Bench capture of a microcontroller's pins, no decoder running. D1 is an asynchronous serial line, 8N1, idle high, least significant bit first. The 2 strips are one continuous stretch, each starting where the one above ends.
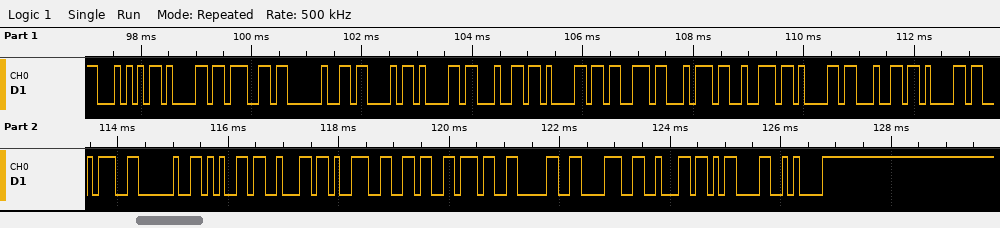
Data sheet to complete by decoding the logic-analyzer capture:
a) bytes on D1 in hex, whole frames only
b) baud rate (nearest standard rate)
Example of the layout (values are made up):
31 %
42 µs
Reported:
54 61 67 20 43 61 64 61 73 74 72 61 64 61 3A 20 65 62 39 36 37 30 38 62 0D 0A
9600 baud
